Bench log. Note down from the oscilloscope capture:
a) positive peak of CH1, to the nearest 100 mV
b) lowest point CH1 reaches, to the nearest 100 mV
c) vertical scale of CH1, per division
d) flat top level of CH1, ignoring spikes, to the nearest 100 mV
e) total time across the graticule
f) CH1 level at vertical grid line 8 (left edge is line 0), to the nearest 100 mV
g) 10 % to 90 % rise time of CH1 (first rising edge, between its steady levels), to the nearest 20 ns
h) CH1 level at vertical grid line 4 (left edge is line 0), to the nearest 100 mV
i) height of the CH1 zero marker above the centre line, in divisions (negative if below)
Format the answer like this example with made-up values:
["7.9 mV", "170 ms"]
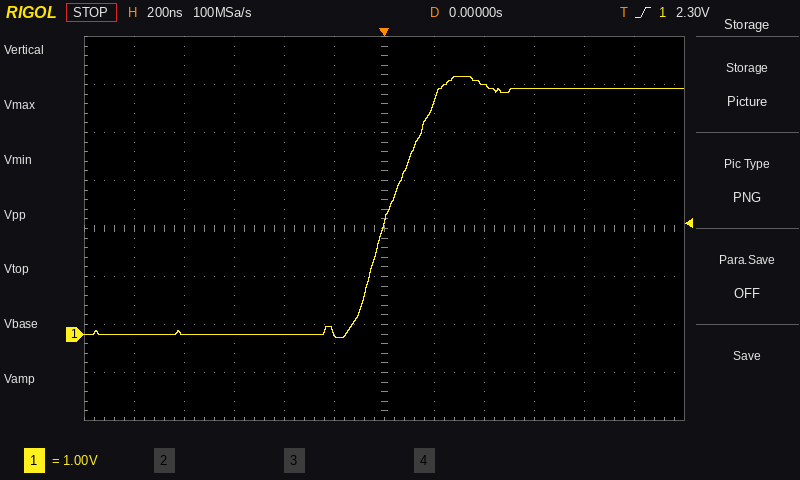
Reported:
["5.4 V", "-100 mV", "1 V", "5.1 V", "2.4 µs", "5.2 V", "280 ns", "0.0 V", "-2.2 div"]
